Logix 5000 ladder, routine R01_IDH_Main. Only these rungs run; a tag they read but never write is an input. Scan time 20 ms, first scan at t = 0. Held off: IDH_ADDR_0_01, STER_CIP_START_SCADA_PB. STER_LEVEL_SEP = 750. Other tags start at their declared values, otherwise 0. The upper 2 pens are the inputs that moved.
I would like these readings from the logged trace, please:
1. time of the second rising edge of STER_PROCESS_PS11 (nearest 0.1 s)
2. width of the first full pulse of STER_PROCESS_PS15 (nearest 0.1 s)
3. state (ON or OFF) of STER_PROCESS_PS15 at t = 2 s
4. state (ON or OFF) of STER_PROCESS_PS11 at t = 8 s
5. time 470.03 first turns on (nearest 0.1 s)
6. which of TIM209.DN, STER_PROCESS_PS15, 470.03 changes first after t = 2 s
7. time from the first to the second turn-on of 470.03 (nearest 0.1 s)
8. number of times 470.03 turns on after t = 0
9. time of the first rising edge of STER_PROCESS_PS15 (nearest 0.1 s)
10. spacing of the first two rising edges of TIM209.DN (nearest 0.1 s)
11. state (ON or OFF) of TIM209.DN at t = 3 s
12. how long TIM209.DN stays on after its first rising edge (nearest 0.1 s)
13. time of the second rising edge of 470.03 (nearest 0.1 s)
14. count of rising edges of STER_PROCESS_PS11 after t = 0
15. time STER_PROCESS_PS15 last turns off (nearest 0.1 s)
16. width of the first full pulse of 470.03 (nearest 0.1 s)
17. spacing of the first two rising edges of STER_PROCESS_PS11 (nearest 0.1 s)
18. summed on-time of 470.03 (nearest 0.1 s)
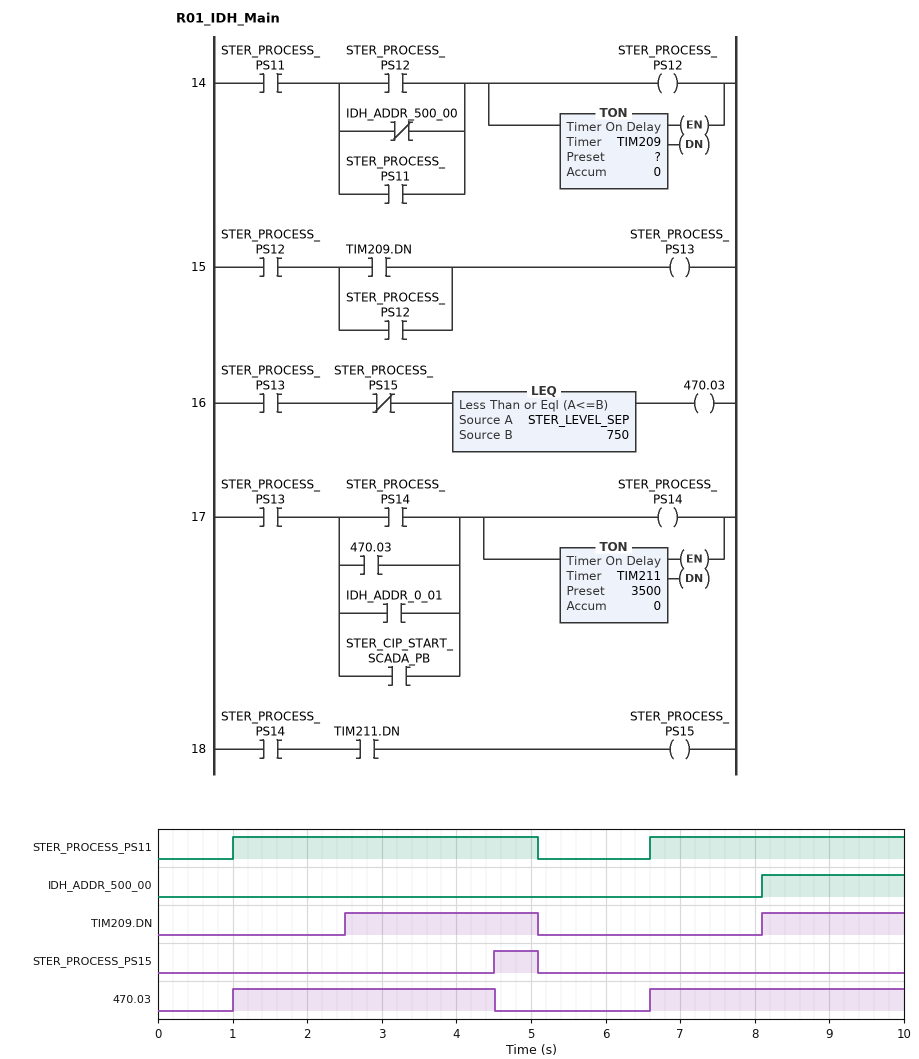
6.6 s
0.6 s
OFF
ON
1.0 s
TIM209.DN
5.6 s
2
4.5 s
5.6 s
ON
2.6 s
6.6 s
2
5.1 s
3.5 s
5.6 s
6.9 s
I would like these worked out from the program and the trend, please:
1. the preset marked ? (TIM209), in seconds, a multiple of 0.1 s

1.5 s
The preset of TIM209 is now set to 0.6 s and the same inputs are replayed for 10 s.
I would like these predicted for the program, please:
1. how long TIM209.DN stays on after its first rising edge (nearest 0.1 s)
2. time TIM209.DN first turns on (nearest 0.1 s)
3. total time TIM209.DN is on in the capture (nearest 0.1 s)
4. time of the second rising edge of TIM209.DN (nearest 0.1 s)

3.5 s
1.6 s
6.3 s
7.2 s
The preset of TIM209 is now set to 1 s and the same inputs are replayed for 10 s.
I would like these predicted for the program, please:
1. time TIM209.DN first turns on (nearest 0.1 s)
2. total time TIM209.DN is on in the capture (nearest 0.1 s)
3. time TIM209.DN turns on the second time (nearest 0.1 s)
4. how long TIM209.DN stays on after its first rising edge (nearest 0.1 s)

2.0 s
5.5 s
7.6 s
3.1 s
